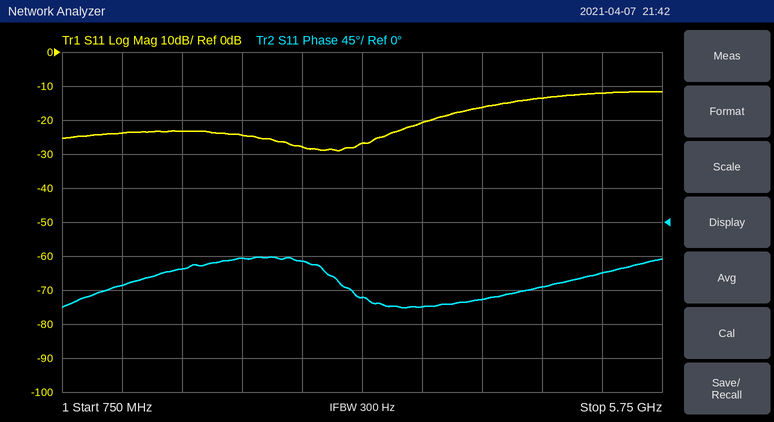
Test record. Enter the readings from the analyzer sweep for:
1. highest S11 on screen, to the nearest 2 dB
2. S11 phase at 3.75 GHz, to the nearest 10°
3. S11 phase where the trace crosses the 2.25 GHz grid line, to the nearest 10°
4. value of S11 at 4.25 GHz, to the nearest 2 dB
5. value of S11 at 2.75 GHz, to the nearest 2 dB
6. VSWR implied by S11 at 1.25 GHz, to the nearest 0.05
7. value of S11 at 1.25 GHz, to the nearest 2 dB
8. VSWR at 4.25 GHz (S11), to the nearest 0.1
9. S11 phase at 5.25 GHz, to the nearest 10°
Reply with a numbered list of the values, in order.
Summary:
1. -12 dB
2. -110°
3. -50°
4. -16 dB
5. -28 dB
6. 1.15
7. -24 dB
8. 1.4
9. -70°
